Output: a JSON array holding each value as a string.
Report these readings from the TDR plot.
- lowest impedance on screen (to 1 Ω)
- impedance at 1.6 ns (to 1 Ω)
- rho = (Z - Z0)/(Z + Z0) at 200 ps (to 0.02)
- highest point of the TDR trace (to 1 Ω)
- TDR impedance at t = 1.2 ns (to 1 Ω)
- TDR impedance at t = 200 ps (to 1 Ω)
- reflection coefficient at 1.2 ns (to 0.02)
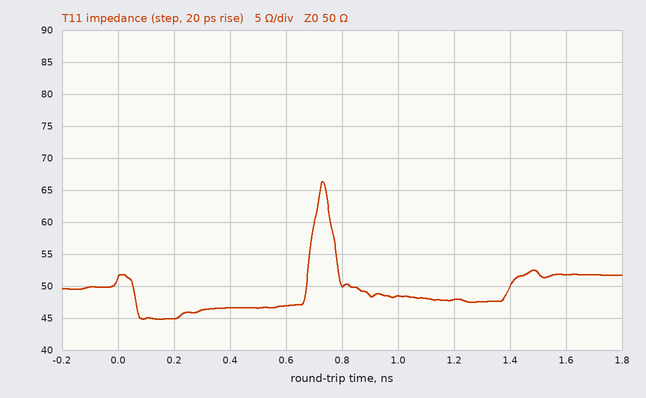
["45 Ω", "52 Ω", "-0.06", "66 Ω", "48 Ω", "45 Ω", "-0.02"]
